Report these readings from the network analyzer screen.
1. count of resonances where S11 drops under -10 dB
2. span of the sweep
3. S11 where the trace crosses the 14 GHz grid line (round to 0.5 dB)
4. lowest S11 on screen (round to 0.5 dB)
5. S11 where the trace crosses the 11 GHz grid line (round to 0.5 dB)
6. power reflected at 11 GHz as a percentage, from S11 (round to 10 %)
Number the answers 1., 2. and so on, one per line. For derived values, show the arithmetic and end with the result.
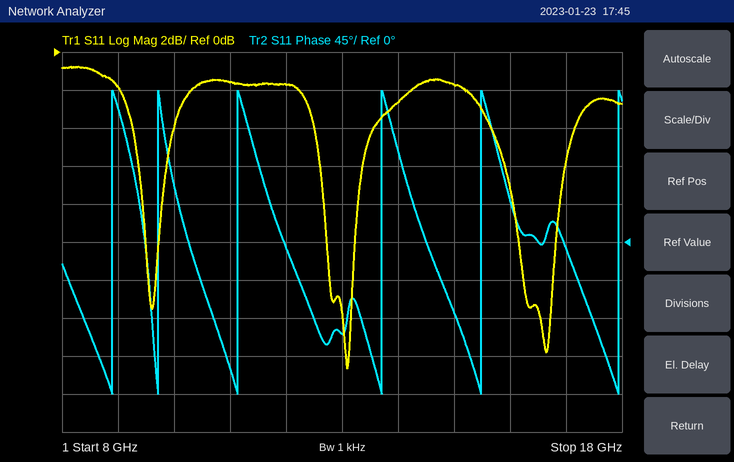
1. 3
2. 10 GHz
3. -2.5 dB
4. -16.5 dB
5. -1.5 dB
6. 10^(-1.5/10) ≈ 70.8 %, so 70 % to the nearest 10 %
